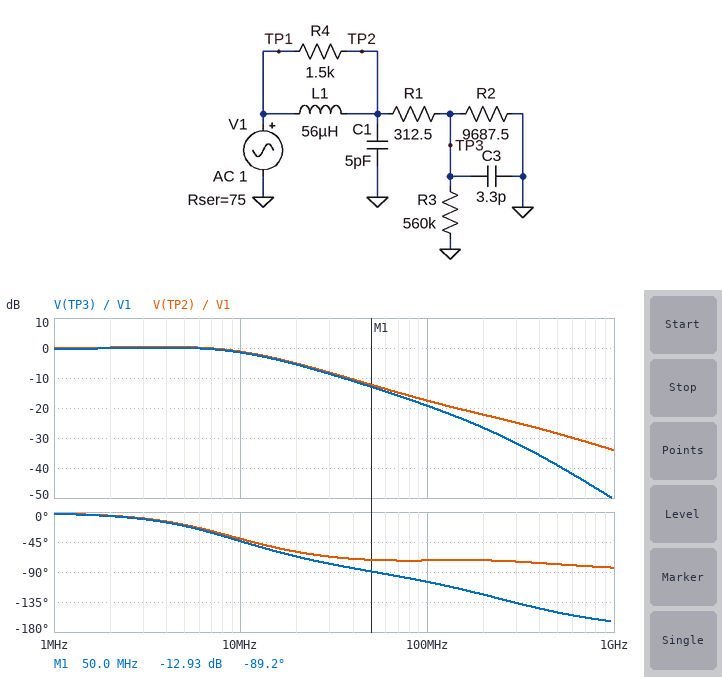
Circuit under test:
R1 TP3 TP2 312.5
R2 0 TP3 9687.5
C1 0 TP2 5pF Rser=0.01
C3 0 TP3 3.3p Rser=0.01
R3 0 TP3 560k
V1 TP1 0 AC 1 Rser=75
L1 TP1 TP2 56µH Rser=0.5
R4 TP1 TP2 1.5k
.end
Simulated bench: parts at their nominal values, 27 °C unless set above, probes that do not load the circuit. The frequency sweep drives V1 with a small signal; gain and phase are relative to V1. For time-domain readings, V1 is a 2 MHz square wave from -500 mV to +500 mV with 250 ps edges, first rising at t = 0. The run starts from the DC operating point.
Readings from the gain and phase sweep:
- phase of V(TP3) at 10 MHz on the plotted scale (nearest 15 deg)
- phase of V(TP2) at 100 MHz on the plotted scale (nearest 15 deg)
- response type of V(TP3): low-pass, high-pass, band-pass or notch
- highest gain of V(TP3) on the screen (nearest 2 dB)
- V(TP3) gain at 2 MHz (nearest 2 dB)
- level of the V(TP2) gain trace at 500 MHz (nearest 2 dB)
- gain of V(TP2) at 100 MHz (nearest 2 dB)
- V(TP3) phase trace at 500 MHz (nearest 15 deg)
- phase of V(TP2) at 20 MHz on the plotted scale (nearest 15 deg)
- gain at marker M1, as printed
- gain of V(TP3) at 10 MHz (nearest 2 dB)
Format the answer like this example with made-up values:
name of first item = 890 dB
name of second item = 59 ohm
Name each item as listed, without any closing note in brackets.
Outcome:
phase of V(TP3) at 10 MHz on the plotted scale = -45 deg
phase of V(TP2) at 100 MHz on the plotted scale = -75 deg
response type of V(TP3): low-pass, high-pass, band-pass or notch = low-pass
highest gain of V(TP3) on the screen = 0 dB
V(TP3) gain at 2 MHz = 0 dB
level of the V(TP2) gain trace at 500 MHz = -28 dB
gain of V(TP2) at 100 MHz = -18 dB
V(TP3) phase trace at 500 MHz = -150 deg
phase of V(TP2) at 20 MHz on the plotted scale = -60 deg
gain at marker M1, as printed = -12.93 dB
gain of V(TP3) at 10 MHz = -2 dB
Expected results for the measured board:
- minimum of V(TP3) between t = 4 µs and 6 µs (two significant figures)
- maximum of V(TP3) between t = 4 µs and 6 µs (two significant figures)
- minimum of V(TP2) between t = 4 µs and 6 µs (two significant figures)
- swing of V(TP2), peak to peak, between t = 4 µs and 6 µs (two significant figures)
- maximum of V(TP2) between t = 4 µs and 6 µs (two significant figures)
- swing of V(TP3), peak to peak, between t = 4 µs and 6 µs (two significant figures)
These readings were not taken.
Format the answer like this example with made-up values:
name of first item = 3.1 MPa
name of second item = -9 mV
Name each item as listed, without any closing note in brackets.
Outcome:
minimum of V(TP3) between t = 4 µs and 6 µs = -540 mV
maximum of V(TP3) between t = 4 µs and 6 µs = 540 mV
minimum of V(TP2) between t = 4 µs and 6 µs = -560 mV
swing of V(TP2), peak to peak, between t = 4 µs and 6 µs = 1.1 V
maximum of V(TP2) between t = 4 µs and 6 µs = 560 mV
swing of V(TP3), peak to peak, between t = 4 µs and 6 µs = 1.1 V
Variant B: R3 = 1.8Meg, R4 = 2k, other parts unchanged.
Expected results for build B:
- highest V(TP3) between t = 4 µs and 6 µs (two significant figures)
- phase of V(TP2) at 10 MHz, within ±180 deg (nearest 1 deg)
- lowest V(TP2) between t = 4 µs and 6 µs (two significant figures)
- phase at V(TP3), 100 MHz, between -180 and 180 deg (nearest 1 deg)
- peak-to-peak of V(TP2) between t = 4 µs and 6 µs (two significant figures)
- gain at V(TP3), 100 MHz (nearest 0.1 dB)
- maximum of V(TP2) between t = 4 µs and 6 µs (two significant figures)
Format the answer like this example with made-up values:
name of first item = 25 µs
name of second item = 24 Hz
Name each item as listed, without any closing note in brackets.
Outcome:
highest V(TP3) between t = 4 µs and 6 µs = 580 mV
phase of V(TP2) at 10 MHz, within ±180 deg = -51 deg
lowest V(TP2) between t = 4 µs and 6 µs = -600 mV
phase at V(TP3), 100 MHz, between -180 and 180 deg = -107 deg
peak-to-peak of V(TP2) between t = 4 µs and 6 µs = 1.2 V
gain at V(TP3), 100 MHz = -21.6 dB
maximum of V(TP2) between t = 4 µs and 6 µs = 600 mV
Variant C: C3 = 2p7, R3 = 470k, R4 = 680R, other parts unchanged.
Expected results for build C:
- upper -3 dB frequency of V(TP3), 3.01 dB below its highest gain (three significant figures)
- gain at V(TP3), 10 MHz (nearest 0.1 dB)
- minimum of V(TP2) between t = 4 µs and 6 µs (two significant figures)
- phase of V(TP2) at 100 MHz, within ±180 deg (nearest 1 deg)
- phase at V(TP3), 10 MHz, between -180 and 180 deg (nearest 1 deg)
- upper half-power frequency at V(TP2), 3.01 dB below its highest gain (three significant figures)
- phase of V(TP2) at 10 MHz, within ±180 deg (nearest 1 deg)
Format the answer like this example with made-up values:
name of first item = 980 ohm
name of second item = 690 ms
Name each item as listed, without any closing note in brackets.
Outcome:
upper -3 dB frequency of V(TP3), 3.01 dB below its highest gain = 26.3 MHz
gain at V(TP3), 10 MHz = -1.0 dB
minimum of V(TP2) between t = 4 µs and 6 µs = -500 mV
phase of V(TP2) at 100 MHz, within ±180 deg = -66 deg
phase at V(TP3), 10 MHz, between -180 and 180 deg = -22 deg
upper half-power frequency at V(TP2), 3.01 dB below its highest gain = 26.8 MHz
phase of V(TP2) at 10 MHz, within ±180 deg = -19 deg
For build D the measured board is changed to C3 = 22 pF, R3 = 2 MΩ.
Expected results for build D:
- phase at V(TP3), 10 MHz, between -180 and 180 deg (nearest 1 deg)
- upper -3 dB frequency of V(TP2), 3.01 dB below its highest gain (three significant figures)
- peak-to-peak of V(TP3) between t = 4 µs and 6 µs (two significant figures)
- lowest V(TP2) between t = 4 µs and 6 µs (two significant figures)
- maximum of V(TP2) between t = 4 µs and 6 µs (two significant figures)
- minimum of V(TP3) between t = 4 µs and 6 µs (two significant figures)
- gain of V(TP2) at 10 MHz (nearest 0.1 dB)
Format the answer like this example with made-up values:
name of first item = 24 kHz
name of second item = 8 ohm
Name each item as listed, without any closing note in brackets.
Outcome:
phase at V(TP3), 10 MHz, between -180 and 180 deg = -89 deg
upper -3 dB frequency of V(TP2), 3.01 dB below its highest gain = 5.32 MHz
peak-to-peak of V(TP3) between t = 4 µs and 6 µs = 1.3 V
lowest V(TP2) between t = 4 µs and 6 µs = -670 mV
maximum of V(TP2) between t = 4 µs and 6 µs = 670 mV
minimum of V(TP3) between t = 4 µs and 6 µs = -640 mV
gain of V(TP2) at 10 MHz = -7.7 dB
